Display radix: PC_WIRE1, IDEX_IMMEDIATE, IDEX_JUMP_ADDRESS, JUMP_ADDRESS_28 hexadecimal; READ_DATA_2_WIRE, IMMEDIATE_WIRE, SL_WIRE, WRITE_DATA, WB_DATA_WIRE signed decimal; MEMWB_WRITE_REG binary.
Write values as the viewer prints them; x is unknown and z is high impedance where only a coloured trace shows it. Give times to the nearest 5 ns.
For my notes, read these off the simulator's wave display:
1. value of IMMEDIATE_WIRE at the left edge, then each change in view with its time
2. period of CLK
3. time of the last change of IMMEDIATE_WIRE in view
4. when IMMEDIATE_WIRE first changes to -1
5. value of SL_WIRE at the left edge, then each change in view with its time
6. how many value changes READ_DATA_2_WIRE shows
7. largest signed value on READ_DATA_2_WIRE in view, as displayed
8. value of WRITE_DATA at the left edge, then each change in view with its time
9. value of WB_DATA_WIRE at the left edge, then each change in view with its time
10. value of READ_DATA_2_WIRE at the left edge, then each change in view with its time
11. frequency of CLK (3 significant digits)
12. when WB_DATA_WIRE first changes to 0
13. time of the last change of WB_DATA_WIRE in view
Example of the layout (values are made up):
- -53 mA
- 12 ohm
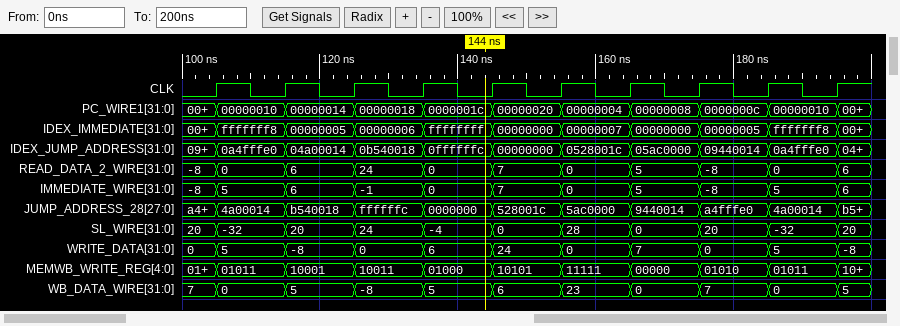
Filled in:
- -8, 5 at 105 ns, 6 at 115 ns, -1 at 125 ns, 0 at 135 ns, 7 at 145 ns, 0 at 155 ns, 5 at 165 ns, -8 at 175 ns, 5 at 185 ns, 6 at 195 ns
- 10 ns
- 195 ns
- 125 ns
- 20, -32 at 105 ns, 20 at 115 ns, 24 at 125 ns, -4 at 135 ns, 0 at 145 ns, 28 at 155 ns, 0 at 165 ns, 20 at 175 ns, -32 at 185 ns, 20 at 195 ns
- 10
- 24
- 0, 5 at 105 ns, -8 at 115 ns, 0 at 125 ns, 6 at 135 ns, 24 at 145 ns, 0 at 155 ns, 7 at 165 ns, 0 at 175 ns, 5 at 185 ns, -8 at 195 ns
- 7, 0 at 105 ns, 5 at 115 ns, -8 at 125 ns, 5 at 135 ns, 6 at 145 ns, 23 at 155 ns, 0 at 165 ns, 7 at 175 ns, 0 at 185 ns, 5 at 195 ns
- -8, 0 at 105 ns, 6 at 115 ns, 24 at 125 ns, 0 at 135 ns, 7 at 145 ns, 0 at 155 ns, 5 at 165 ns, -8 at 175 ns, 0 at 185 ns, 6 at 195 ns
- 100 MHz
- 105 ns
- 195 ns
